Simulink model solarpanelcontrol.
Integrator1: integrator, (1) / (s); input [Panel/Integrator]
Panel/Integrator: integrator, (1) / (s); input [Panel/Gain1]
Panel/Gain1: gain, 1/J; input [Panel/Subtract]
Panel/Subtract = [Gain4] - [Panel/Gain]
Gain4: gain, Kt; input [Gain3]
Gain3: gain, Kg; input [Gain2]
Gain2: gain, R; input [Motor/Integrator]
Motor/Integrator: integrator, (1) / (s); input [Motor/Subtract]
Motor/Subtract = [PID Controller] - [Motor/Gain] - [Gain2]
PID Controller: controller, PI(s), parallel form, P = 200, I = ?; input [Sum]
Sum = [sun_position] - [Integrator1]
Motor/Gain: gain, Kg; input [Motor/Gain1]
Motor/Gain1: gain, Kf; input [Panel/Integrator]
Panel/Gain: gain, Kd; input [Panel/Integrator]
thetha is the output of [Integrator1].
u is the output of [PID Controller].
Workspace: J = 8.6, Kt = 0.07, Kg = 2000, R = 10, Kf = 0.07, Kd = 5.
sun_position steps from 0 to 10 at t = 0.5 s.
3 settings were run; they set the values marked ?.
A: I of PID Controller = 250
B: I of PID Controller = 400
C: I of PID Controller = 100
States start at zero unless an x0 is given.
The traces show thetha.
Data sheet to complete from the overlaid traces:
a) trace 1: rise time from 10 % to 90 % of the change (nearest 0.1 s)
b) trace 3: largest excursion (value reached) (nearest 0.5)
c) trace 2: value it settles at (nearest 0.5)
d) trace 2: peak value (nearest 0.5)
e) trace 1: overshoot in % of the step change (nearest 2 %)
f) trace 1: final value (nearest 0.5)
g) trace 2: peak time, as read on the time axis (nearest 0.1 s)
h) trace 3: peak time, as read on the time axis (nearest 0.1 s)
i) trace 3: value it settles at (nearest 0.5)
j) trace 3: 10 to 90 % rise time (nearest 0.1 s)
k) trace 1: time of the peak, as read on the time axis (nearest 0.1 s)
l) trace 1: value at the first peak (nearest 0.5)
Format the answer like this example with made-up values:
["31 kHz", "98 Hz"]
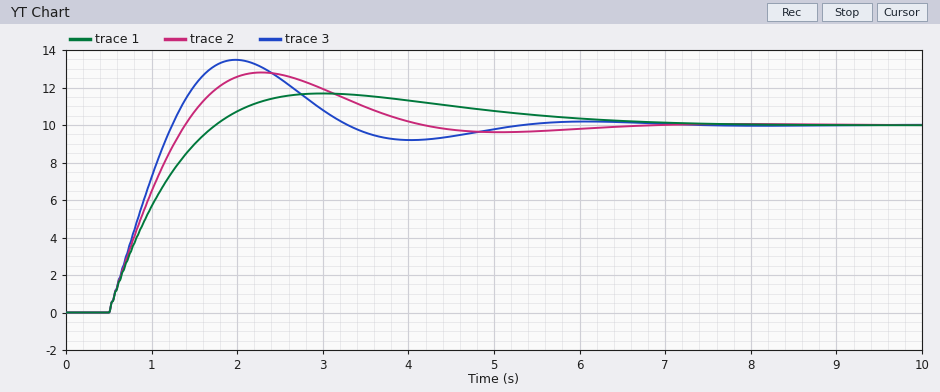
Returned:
["0.9 s", "13.5", "10.0", "13.0", "16 %", "10.0", "2.3 s", "2.0 s", "10.0", "0.6 s", "3.0 s", "11.5"]
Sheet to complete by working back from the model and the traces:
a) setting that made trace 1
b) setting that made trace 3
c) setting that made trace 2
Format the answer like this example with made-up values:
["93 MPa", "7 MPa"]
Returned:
["C", "B", "A"]
